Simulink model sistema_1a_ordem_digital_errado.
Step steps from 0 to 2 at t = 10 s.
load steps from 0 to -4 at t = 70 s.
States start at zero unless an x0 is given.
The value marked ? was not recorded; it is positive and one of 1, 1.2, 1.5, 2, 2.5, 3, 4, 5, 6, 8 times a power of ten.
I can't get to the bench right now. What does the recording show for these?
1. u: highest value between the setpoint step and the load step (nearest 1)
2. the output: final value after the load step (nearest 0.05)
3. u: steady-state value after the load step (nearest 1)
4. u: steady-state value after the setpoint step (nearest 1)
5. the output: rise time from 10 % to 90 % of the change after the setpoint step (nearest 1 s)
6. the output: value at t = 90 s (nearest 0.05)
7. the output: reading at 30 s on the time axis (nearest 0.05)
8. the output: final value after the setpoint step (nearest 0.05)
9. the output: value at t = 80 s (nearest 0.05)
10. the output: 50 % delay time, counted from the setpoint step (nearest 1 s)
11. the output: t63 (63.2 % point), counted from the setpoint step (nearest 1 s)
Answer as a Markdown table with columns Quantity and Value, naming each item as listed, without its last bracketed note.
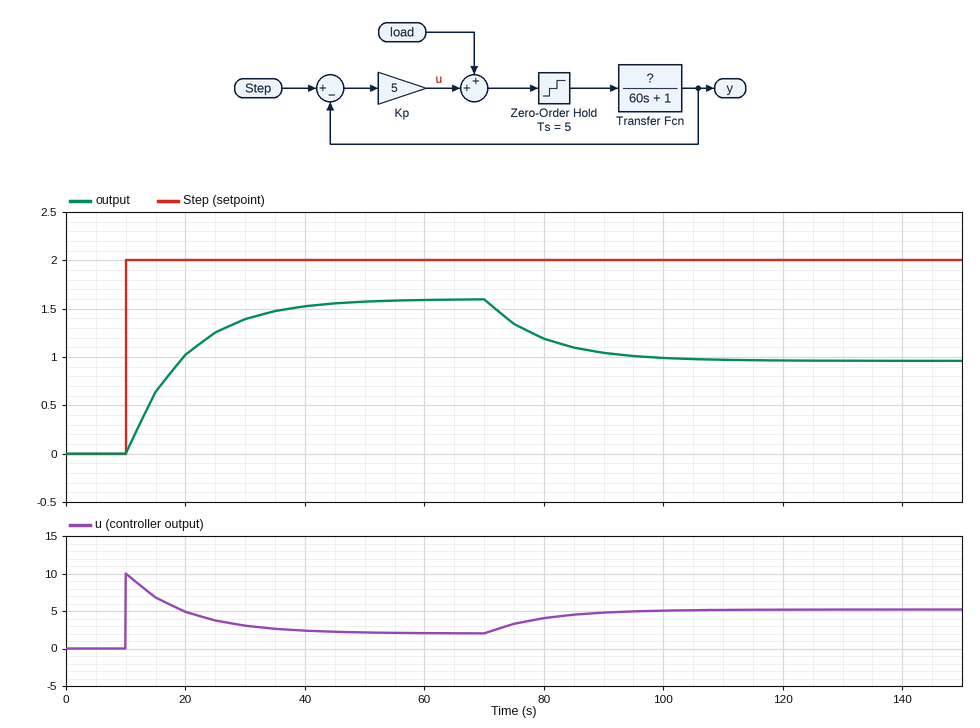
| Quantity | Value |
|---|---|
| u: highest value between the setpoint step and the load step | 10 |
| the output: final value after the load step | 0.95 |
| u: steady-state value after the load step | 5 |
| u: steady-state value after the setpoint step | 2 |
| the output: rise time from 10 % to 90 % of the change after the setpoint step | 22 s |
| the output: value at t = 90 s | 1.05 |
| the output: reading at 30 s on the time axis | 1.40 |
| the output: final value after the setpoint step | 1.60 |
| the output: value at t = 80 s | 1.20 |
| the output: 50 % delay time, counted from the setpoint step | 7 s |
| the output: t63 (63.2 % point), counted from the setpoint step | 10 s |
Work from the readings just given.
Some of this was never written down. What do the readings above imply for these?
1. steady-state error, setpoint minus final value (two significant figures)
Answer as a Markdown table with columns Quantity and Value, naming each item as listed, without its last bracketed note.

| Quantity | Value |
|---|---|
| steady-state error, setpoint minus final value | 0.40 |
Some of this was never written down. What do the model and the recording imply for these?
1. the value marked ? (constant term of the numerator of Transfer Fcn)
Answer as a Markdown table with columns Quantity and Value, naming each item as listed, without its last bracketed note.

| Quantity | Value |
|---|---|
| the value marked ? | 0.8 |
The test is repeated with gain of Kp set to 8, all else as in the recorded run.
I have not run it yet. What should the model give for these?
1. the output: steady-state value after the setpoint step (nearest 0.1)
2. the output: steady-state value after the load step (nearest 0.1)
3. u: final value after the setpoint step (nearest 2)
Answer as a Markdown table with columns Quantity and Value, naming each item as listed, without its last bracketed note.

| Quantity | Value |
|---|---|
| the output: steady-state value after the setpoint step | 1.7 |
| the output: steady-state value after the load step | 1.3 |
| u: final value after the setpoint step | 2 |
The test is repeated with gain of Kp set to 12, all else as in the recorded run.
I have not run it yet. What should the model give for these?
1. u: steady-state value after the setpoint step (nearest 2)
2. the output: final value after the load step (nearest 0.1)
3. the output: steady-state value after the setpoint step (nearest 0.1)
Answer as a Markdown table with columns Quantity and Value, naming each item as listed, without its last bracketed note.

| Quantity | Value |
|---|---|
| u: steady-state value after the setpoint step | 2 |
| the output: final value after the load step | 1.5 |
| the output: steady-state value after the setpoint step | 1.8 |
